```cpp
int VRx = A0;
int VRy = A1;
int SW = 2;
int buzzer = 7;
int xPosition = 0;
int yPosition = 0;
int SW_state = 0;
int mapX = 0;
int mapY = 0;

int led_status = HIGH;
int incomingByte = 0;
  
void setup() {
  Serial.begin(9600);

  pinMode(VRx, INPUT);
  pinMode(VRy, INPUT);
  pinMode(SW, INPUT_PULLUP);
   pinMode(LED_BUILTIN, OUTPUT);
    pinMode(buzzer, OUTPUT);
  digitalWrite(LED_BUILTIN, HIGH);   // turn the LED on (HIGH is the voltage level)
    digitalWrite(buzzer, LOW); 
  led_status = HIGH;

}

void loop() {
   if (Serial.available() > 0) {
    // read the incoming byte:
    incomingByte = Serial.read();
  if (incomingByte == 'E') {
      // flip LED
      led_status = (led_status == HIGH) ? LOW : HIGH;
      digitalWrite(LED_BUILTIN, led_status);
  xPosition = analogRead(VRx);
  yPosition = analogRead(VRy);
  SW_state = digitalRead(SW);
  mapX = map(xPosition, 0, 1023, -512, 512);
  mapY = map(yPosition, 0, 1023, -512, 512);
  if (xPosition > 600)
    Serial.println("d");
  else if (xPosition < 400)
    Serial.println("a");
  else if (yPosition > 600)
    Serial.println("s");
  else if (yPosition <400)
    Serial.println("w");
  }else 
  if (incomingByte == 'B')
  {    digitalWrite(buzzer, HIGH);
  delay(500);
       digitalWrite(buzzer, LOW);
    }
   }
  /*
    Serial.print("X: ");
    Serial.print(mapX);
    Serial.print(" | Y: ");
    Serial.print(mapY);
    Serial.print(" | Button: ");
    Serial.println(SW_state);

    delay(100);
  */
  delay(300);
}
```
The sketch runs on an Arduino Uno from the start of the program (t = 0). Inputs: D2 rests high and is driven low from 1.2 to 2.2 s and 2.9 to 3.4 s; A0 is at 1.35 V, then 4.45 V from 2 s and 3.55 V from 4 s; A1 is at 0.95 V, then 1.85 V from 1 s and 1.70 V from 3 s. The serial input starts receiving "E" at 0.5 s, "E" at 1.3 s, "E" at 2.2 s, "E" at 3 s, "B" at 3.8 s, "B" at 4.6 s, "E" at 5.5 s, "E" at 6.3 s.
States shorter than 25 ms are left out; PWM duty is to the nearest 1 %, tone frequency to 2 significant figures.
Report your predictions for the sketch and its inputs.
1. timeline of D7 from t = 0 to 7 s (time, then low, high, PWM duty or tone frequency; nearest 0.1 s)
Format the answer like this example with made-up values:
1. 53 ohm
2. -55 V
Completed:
1. 0 s low; 3.9 s high; 4.4 s low; 4.7 s high; 5.2 s low
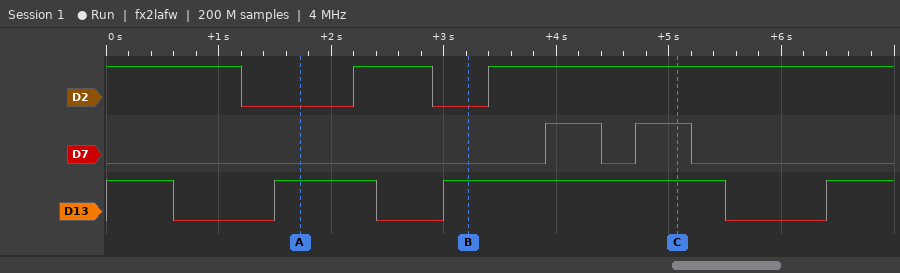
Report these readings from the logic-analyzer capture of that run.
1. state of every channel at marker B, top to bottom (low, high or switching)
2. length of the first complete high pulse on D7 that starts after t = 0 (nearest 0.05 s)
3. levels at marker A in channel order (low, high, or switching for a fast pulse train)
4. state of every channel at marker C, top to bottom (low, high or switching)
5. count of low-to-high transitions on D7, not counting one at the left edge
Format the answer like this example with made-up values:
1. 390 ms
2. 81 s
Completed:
1. D2 low, D7 low, D13 high
2. 0.50 s
3. D2 low, D7 low, D13 high
4. D2 high, D7 high, D13 high
5. 2
